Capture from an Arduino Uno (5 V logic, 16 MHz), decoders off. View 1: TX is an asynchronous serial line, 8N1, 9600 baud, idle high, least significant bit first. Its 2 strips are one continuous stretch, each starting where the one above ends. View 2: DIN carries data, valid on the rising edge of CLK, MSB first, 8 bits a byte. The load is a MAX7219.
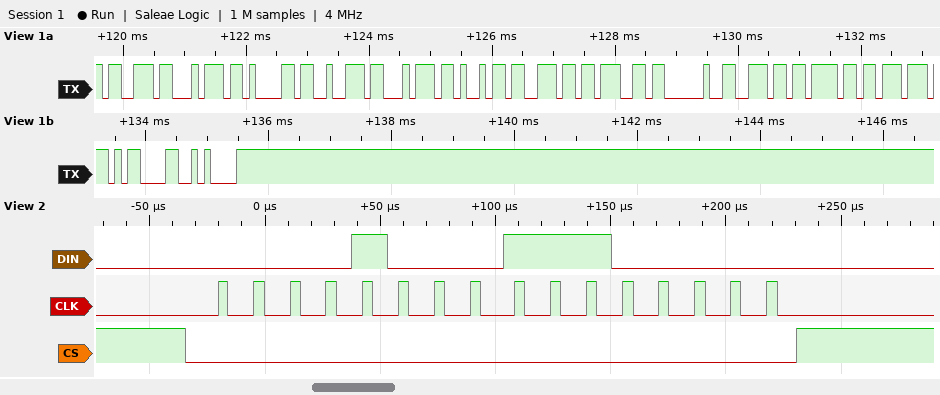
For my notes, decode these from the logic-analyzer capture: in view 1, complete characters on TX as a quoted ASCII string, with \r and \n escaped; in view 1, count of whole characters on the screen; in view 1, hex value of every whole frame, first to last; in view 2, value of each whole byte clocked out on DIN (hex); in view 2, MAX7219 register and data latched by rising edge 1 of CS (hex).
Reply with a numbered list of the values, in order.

1. "starting now\r\n"
2. 14
3. 0x73 0x74 0x61 0x72 0x74 0x69 0x6E 0x67 0x20 0x6E 0x6F 0x77 0x0D 0x0A
4. 08 E0
5. register 0x8, data 0xE0
